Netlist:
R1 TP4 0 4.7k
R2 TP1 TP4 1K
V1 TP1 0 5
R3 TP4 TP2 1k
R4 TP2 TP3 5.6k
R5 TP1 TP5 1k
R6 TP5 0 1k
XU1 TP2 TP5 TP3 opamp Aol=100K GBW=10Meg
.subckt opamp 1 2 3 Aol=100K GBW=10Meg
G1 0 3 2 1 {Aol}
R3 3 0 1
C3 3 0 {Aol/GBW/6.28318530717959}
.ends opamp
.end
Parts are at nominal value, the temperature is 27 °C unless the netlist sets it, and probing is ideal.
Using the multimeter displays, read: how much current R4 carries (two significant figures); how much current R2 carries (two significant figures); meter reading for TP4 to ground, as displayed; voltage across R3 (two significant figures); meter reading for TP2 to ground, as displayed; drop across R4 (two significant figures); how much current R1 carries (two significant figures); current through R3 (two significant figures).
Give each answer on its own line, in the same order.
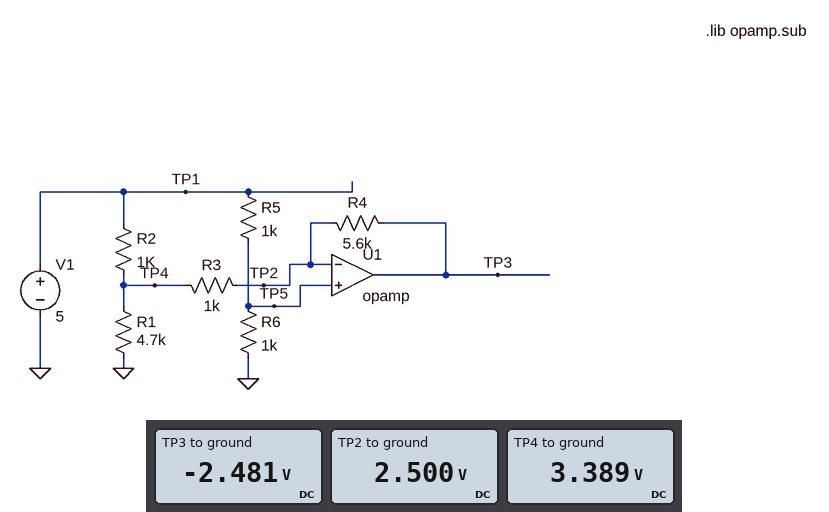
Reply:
890 µA
1.6 mA
3.389 V
890 mV
2.500 V
5.0 V
720 µA
890 µA
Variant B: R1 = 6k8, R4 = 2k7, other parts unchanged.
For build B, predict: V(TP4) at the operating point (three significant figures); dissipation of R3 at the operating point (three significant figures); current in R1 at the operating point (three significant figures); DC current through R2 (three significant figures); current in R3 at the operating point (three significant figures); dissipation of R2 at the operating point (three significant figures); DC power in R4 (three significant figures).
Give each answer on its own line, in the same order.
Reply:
3.49 V
986 µW
514 µA
1.51 mA
993 µA
2.27 mW
2.66 mW
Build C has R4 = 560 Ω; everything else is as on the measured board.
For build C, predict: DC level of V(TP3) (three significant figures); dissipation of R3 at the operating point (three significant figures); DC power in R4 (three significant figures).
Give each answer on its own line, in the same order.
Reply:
2.00 V
791 µW
443 µW
